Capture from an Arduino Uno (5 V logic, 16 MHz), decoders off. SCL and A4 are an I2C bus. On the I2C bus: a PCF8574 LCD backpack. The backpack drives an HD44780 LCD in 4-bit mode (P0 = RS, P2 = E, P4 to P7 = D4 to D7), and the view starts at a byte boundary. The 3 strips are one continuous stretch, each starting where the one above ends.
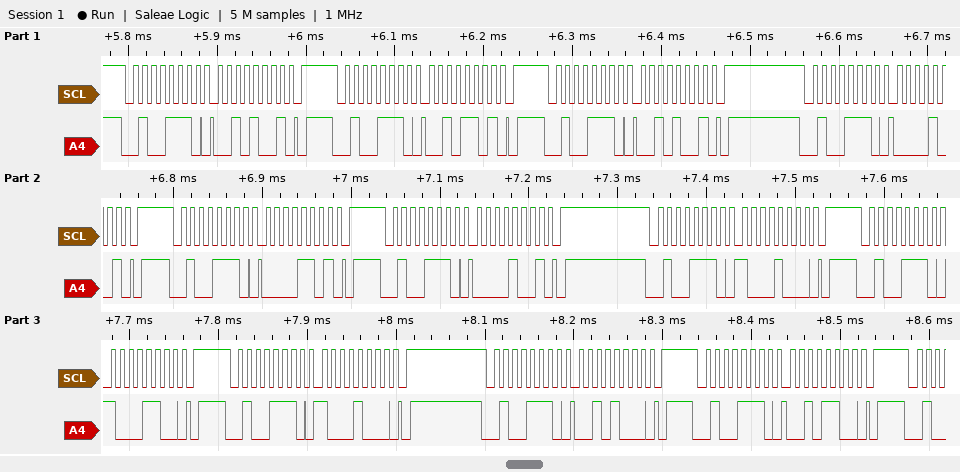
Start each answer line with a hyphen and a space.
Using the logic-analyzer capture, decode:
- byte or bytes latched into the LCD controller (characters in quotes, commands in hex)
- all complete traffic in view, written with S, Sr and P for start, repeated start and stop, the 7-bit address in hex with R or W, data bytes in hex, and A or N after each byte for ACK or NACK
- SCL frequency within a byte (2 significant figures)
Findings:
- ' '
- S 27W A 29 A P S 27W A 2D A P S 27W A 29 A P S 27W A 09 A P S 27W A 0D A P S 27W A 09 A P S 27W A 88 A P S 27W A 8C A P S 27W A 88 A P S 27W A 28 A P S 27W A 2C A P
- 100 kHz
